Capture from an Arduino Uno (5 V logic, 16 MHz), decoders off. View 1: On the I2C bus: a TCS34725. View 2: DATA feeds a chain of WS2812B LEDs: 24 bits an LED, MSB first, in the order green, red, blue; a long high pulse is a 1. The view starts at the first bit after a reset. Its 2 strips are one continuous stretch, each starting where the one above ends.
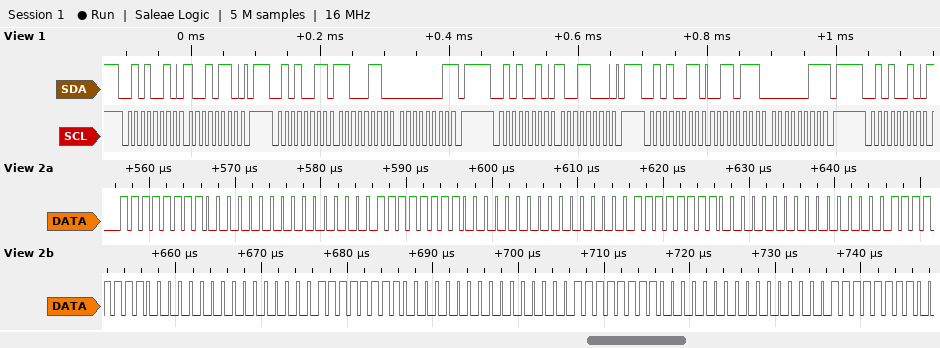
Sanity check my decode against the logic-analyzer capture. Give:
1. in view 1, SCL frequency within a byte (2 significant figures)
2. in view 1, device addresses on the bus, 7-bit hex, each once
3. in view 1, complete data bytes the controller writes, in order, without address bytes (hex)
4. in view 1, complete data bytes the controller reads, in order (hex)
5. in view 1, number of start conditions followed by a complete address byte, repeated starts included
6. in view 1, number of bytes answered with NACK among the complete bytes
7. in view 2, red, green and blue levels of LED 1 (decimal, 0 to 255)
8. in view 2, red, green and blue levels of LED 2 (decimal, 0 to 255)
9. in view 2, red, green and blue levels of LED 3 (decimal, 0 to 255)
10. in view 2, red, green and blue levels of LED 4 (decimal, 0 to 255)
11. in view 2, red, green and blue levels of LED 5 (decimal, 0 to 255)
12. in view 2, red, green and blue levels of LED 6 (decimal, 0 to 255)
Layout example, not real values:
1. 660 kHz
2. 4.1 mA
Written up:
1. 100 kHz
2. 0x29
3. 96 98
4. C6 01 37 03
5. 5
6. 2
7. 0, 255, 0
8. 0, 255, 0
9. 0, 255, 0
10. 0, 255, 0
11. 0, 255, 0
12. 0, 255, 0
